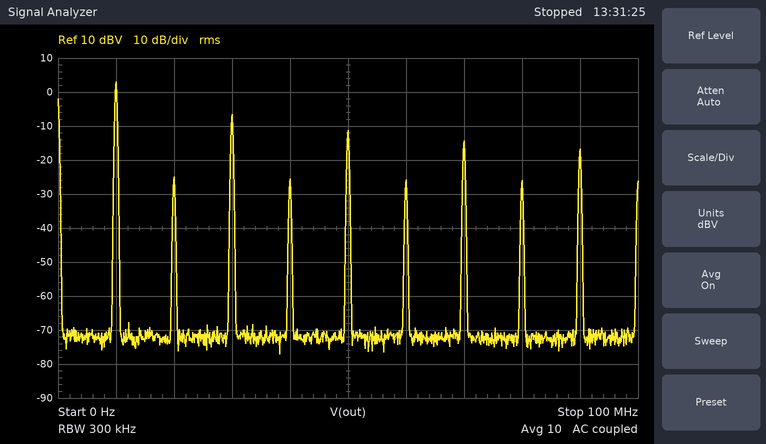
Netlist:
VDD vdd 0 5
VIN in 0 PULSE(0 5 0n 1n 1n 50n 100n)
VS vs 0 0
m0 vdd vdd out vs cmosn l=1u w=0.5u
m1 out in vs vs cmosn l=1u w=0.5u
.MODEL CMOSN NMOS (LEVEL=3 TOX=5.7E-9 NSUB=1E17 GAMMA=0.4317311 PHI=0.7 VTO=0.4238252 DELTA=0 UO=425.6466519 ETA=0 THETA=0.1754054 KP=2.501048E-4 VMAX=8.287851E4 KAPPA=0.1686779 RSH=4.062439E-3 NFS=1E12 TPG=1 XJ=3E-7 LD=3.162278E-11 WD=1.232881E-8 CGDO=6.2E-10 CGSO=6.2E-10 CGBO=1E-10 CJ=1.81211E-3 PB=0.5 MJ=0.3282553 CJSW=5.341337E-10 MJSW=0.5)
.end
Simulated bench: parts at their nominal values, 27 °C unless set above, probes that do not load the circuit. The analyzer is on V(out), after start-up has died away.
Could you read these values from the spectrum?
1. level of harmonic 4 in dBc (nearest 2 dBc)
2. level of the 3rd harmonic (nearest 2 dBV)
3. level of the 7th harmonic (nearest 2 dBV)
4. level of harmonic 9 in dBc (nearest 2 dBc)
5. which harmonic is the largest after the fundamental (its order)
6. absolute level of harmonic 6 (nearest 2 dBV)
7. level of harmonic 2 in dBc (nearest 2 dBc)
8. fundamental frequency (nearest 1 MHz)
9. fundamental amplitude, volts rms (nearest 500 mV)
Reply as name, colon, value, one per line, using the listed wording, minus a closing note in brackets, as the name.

level of harmonic 4 in dBc: -28 dBc
level of the 3rd harmonic: -6 dBV
level of the 7th harmonic: -14 dBV
level of harmonic 9 in dBc: -20 dBc
which harmonic is the largest after the fundamental: 3
absolute level of harmonic 6: -26 dBV
level of harmonic 2 in dBc: -28 dBc
fundamental frequency: 10 MHz
fundamental amplitude, volts rms: 1.5 V
